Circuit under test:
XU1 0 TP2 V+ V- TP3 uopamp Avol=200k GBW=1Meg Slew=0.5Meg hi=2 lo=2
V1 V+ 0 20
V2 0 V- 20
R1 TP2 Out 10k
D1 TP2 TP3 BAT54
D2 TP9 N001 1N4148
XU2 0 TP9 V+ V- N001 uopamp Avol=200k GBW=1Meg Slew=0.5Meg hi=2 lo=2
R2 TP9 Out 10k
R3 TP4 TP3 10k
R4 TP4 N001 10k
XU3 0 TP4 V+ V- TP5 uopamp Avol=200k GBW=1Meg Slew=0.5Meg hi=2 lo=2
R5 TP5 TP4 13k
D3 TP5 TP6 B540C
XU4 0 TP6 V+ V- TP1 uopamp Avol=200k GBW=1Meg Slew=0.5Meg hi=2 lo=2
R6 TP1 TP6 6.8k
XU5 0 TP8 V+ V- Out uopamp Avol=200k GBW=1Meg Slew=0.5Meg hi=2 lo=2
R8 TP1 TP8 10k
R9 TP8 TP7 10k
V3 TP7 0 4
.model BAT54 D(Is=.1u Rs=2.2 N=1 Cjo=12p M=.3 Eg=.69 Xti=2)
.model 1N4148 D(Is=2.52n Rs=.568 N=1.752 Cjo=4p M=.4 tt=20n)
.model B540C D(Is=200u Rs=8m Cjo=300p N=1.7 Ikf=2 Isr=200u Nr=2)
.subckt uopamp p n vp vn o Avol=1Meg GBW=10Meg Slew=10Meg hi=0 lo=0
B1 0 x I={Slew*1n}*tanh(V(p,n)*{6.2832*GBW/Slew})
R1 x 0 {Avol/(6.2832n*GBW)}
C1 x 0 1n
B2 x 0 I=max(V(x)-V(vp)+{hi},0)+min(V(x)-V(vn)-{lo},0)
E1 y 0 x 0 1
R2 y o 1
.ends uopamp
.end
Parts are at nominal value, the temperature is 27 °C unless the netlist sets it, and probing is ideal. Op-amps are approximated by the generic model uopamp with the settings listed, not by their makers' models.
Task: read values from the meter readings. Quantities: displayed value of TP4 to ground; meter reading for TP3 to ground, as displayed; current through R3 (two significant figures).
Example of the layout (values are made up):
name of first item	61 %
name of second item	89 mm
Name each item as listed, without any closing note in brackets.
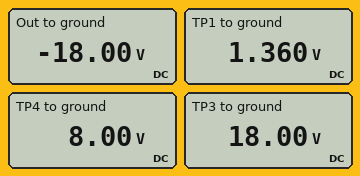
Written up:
displayed value of TP4 to ground	8.00 V
meter reading for TP3 to ground, as displayed	18.00 V
current through R3	1.0 mA
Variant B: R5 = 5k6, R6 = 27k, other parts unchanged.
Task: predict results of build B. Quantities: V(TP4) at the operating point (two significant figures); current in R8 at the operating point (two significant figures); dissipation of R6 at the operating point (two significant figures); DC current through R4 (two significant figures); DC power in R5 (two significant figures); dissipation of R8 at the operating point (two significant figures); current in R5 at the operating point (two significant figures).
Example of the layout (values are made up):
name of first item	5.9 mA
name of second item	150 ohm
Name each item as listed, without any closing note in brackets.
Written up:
V(TP4) at the operating point	1.0 V
current in R8 at the operating point	70 µA
dissipation of R6 at the operating point	1.1 mW
DC current through R4	1.7 mA
DC power in R5	65 mW
dissipation of R8 at the operating point	49 µW
current in R5 at the operating point	3.4 mA
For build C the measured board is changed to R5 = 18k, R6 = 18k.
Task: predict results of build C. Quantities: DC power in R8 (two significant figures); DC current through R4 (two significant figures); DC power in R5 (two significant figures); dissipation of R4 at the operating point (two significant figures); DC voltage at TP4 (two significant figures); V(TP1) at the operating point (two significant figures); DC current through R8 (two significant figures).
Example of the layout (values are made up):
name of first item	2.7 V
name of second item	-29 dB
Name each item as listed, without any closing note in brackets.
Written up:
DC power in R8	4.0 µW
DC current through R4	780 µA
DC power in R5	44 mW
dissipation of R4 at the operating point	6.1 mW
DC voltage at TP4	10 V
V(TP1) at the operating point	3.6 V
DC current through R8	20 µA
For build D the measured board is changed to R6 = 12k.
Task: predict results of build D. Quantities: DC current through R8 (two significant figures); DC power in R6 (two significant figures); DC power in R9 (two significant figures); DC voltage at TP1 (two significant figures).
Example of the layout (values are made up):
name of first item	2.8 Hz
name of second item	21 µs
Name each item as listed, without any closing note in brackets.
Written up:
DC current through R8	80 µA
DC power in R6	480 µW
DC power in R9	64 µW
DC voltage at TP1	2.4 V
